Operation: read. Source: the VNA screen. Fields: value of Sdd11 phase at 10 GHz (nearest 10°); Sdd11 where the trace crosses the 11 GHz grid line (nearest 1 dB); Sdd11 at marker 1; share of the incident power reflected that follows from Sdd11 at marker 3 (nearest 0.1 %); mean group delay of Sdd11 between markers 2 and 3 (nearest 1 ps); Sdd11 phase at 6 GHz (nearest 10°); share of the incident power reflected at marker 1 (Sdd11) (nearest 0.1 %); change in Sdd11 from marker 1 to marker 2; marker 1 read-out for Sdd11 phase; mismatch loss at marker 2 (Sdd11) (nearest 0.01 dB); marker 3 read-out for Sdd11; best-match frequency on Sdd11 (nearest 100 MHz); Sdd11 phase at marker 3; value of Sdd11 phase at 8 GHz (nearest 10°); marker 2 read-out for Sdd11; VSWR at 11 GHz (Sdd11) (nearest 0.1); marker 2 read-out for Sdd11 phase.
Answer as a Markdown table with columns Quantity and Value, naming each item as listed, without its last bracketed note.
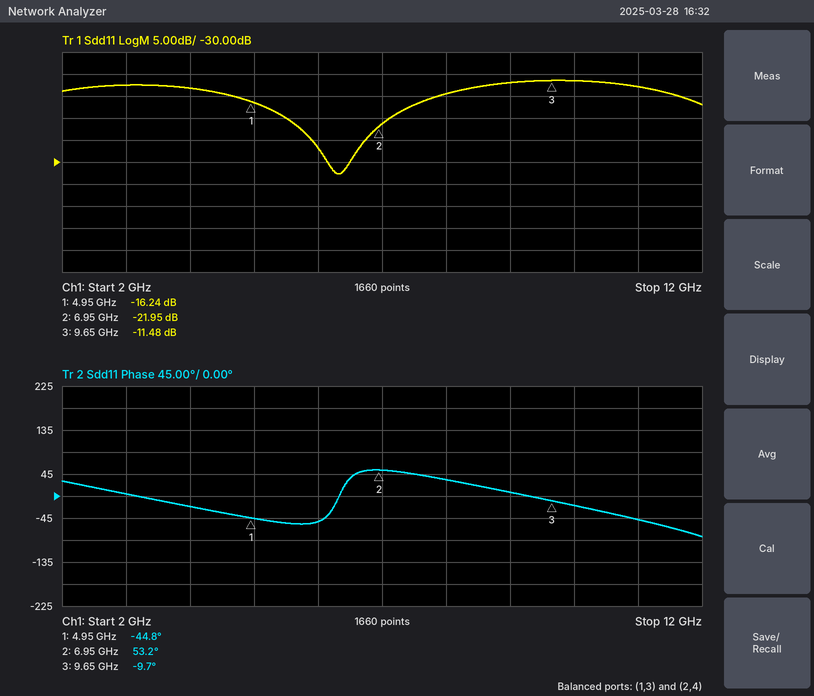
| Quantity | Value |
|---|---|
| value of Sdd11 phase at 10 GHz | -20° |
| Sdd11 where the trace crosses the 11 GHz grid line | -13 dB |
| Sdd11 at marker 1 | -16.24 dB |
| share of the incident power reflected that follows from Sdd11 at marker 3 | 7.1 % |
| mean group delay of Sdd11 between markers 2 and 3 | 65 ps |
| Sdd11 phase at 6 GHz | -50° |
| share of the incident power reflected at marker 1 (Sdd11) | 2.4 % |
| change in Sdd11 from marker 1 to marker 2 | -5.71 dB |
| marker 1 read-out for Sdd11 phase | -44.8° |
| mismatch loss at marker 2 (Sdd11) | 0.03 dB |
| marker 3 read-out for Sdd11 | -11.48 dB |
| best-match frequency on Sdd11 | 6.3 GHz |
| Sdd11 phase at marker 3 | -9.7° |
| value of Sdd11 phase at 8 GHz | 30° |
| marker 2 read-out for Sdd11 | -21.95 dB |
| VSWR at 11 GHz (Sdd11) | 1.6 |
| marker 2 read-out for Sdd11 phase | 53.2° |
